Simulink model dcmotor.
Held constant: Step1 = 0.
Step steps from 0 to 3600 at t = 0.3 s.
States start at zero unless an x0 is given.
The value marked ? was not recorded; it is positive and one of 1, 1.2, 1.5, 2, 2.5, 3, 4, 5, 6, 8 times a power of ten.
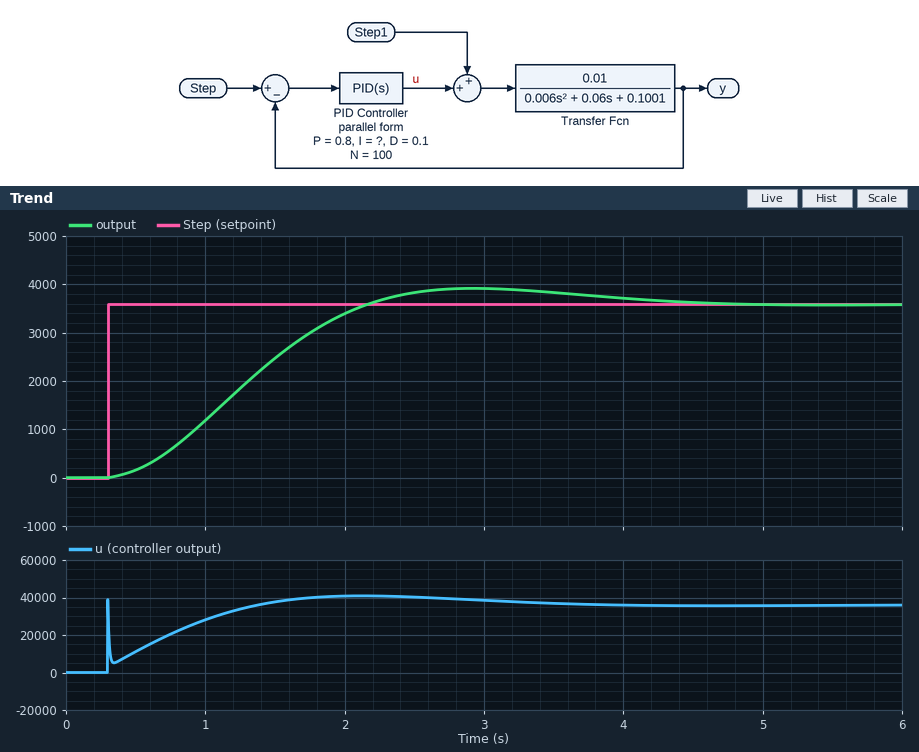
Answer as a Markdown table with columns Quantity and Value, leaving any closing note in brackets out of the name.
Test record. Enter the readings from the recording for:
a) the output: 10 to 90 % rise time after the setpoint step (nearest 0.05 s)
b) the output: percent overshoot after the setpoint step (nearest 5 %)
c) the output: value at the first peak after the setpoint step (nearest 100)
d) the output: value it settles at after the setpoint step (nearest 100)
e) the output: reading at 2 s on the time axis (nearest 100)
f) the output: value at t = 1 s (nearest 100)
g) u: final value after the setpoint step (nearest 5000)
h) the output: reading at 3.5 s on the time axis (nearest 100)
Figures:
| Quantity | Value |
|---|---|
| the output: 10 to 90 % rise time after the setpoint step | 1.25 s |
| the output: percent overshoot after the setpoint step | 10 % |
| the output: value at the first peak after the setpoint step | 3900 |
| the output: value it settles at after the setpoint step | 3600 |
| the output: reading at 2 s on the time axis | 3400 |
| the output: value at t = 1 s | 1200 |
| u: final value after the setpoint step | 35000 |
| the output: reading at 3.5 s on the time axis | 3800 |
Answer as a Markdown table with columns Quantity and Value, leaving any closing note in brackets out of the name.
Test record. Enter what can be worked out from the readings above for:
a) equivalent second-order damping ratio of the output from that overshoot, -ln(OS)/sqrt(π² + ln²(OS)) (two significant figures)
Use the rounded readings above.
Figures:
| Quantity | Value |
|---|---|
| equivalent second-order damping ratio of the output from that overshoot, -ln(OS)/sqrt(π² + ln²(OS)) | 0.59 |
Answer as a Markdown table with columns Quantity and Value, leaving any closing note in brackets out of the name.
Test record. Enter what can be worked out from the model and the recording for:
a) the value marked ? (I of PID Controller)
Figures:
| Quantity | Value |
|---|---|
| the value marked ? | 12 |
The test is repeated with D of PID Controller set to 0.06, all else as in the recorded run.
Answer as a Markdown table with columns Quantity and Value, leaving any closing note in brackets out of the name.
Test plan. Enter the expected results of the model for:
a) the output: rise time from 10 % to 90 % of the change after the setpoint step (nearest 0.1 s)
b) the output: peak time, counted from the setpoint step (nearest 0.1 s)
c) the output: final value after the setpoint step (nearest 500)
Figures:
| Quantity | Value |
|---|---|
| the output: rise time from 10 % to 90 % of the change after the setpoint step | 1.2 s |
| the output: peak time, counted from the setpoint step | 2.6 s |
| the output: final value after the setpoint step | 3500 |
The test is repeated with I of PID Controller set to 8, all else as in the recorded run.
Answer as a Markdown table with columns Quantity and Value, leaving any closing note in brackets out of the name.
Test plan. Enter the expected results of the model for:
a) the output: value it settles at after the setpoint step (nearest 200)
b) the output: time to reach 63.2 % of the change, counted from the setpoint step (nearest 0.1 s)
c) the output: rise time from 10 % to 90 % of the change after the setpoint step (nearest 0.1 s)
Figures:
| Quantity | Value |
|---|---|
| the output: value it settles at after the setpoint step | 3600 |
| the output: time to reach 63.2 % of the change, counted from the setpoint step | 1.5 s |
| the output: rise time from 10 % to 90 % of the change after the setpoint step | 1.9 s |
